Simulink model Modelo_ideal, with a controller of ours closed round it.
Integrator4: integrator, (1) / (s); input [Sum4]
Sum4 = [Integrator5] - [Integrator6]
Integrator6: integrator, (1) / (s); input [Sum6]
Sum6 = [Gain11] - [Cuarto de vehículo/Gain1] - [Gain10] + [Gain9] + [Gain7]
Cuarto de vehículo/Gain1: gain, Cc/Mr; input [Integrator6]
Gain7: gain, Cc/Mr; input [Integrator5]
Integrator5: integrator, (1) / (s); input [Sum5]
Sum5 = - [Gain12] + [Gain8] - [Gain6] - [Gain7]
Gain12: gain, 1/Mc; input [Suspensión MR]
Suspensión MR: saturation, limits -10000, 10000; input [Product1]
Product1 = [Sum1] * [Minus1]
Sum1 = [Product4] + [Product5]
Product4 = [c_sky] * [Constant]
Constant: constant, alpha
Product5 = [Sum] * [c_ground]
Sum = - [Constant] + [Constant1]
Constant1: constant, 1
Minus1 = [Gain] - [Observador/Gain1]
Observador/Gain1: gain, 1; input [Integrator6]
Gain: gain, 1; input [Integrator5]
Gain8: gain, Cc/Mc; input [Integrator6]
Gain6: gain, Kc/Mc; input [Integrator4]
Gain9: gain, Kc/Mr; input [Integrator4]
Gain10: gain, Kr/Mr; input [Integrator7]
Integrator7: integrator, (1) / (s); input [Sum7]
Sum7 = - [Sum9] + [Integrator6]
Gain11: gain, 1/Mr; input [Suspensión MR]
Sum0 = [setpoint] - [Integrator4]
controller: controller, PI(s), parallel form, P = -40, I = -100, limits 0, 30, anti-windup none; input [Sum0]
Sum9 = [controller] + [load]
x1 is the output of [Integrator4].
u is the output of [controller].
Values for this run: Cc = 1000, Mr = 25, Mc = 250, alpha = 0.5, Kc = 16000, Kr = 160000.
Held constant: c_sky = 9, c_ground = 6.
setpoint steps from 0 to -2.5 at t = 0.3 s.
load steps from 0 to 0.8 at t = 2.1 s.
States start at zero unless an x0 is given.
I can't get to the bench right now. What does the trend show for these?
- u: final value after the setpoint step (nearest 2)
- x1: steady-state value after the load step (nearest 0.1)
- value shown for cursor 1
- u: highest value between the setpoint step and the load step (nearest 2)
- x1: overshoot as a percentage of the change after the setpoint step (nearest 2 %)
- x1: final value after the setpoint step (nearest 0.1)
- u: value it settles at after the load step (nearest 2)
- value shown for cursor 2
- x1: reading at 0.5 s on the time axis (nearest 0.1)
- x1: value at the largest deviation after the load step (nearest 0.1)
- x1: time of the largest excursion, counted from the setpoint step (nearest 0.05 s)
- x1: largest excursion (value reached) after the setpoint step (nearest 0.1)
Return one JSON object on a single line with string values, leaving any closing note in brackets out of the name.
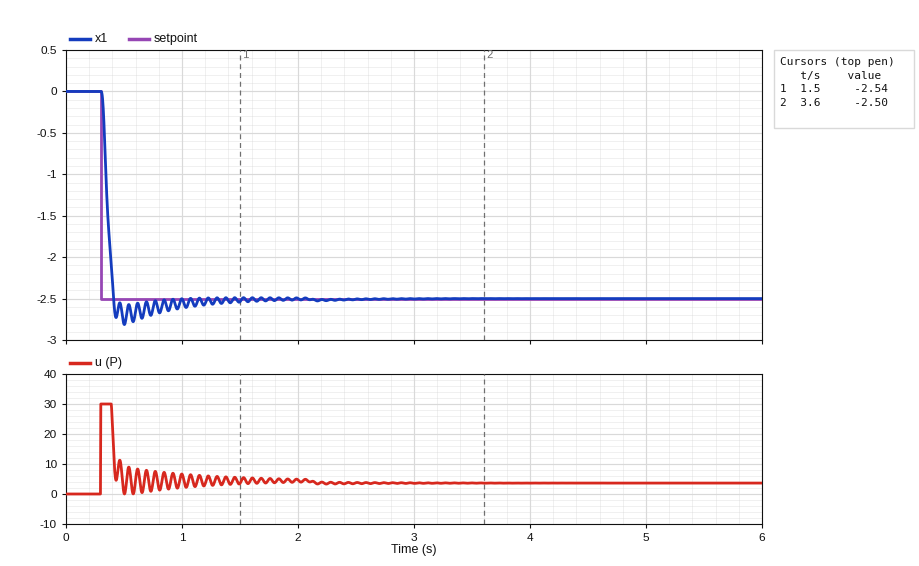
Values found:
{"u: final value after the setpoint step": "4", "x1: steady-state value after the load step": "-2.5", "value shown for cursor 1": "-2.54", "u: highest value between the setpoint step and the load step": "30", "x1: overshoot as a percentage of the change after the setpoint step": "12 %", "x1: final value after the setpoint step": "-2.5", "u: value it settles at after the load step": "4", "value shown for cursor 2": "-2.50", "x1: reading at 0.5 s on the time axis": "-2.8", "x1: value at the largest deviation after the load step": "-2.5", "x1: time of the largest excursion, counted from the setpoint step": "0.20 s", "x1: largest excursion (value reached) after the setpoint step": "-2.8"}
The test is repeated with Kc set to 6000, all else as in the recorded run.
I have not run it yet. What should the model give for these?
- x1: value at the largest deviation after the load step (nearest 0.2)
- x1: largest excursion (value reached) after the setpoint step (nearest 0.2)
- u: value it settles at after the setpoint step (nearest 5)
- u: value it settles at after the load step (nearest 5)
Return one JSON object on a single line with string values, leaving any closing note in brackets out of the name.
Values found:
{"x1: value at the largest deviation after the load step": "-2.6", "x1: largest excursion (value reached) after the setpoint step": "-2.8", "u: value it settles at after the setpoint step": "0", "u: value it settles at after the load step": "0"}
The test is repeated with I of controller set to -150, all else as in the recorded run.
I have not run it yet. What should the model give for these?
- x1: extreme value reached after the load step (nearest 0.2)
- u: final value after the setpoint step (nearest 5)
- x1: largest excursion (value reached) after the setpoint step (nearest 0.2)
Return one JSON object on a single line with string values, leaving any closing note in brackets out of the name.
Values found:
{"x1: extreme value reached after the load step": "-2.6", "u: final value after the setpoint step": "5", "x1: largest excursion (value reached) after the setpoint step": "-3.0"}
